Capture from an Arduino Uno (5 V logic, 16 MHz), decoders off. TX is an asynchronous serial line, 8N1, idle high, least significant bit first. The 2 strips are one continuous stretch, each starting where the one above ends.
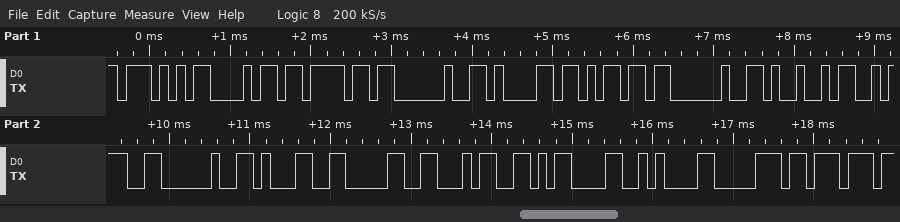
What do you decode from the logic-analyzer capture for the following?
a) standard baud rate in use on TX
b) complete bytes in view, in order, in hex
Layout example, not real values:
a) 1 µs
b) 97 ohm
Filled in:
a) 9600 baud
b) 0x57 0x68 0x6F 0x20 0x61 0x6D 0x20 0x49 0x3A 0x20 0x31 0x30 0x34 0x0D 0x0A 0x70 0x77
